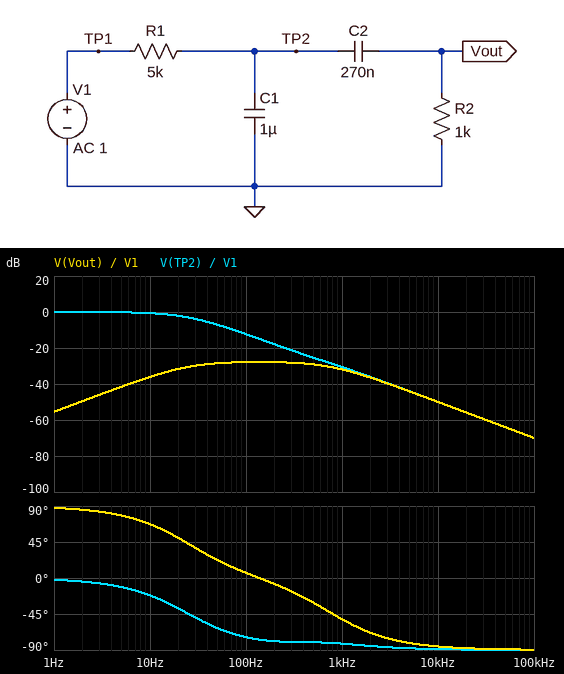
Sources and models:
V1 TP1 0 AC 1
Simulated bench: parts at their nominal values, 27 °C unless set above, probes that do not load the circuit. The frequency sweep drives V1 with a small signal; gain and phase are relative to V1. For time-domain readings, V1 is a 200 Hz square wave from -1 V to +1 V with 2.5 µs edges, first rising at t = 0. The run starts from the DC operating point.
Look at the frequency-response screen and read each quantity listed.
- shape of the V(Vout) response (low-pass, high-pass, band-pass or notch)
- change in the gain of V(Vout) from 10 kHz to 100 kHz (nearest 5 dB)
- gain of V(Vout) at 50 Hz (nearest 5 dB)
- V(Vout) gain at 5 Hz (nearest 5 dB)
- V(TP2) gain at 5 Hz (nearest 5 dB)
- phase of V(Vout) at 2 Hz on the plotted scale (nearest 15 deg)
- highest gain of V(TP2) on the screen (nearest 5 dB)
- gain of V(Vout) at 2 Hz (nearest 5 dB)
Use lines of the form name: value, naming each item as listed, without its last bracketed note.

shape of the V(Vout) response: band-pass
change in the gain of V(Vout) from 10 kHz to 100 kHz: -20 dB
gain of V(Vout) at 50 Hz: -30 dB
V(Vout) gain at 5 Hz: -40 dB
V(TP2) gain at 5 Hz: 0 dB
phase of V(Vout) at 2 Hz on the plotted scale: 90 deg
highest gain of V(TP2) on the screen: 0 dB
gain of V(Vout) at 2 Hz: -50 dB
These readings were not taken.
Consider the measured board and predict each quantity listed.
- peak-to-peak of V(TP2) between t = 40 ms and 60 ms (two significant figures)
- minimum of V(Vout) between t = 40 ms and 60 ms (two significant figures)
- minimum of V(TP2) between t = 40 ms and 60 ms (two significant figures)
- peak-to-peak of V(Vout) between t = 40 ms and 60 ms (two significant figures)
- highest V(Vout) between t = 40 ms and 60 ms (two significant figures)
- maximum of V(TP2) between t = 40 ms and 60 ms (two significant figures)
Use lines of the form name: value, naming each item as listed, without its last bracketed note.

peak-to-peak of V(TP2) between t = 40 ms and 60 ms: 400 mV
minimum of V(Vout) between t = 40 ms and 60 ms: -44 mV
minimum of V(TP2) between t = 40 ms and 60 ms: -200 mV
peak-to-peak of V(Vout) between t = 40 ms and 60 ms: 88 mV
highest V(Vout) between t = 40 ms and 60 ms: 44 mV
maximum of V(TP2) between t = 40 ms and 60 ms: 200 mV
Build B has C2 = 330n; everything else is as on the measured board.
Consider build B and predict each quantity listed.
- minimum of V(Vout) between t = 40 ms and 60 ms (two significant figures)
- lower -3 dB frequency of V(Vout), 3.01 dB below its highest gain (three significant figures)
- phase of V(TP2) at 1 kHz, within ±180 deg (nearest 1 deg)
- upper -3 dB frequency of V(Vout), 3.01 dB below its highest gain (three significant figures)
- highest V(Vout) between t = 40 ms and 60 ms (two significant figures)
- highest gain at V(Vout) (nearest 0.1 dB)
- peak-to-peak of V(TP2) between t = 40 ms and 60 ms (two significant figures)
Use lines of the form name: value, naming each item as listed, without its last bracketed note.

minimum of V(Vout) between t = 40 ms and 60 ms: -50 mV
lower -3 dB frequency of V(Vout), 3.01 dB below its highest gain: 22.1 Hz
phase of V(TP2) at 1 kHz, within ±180 deg: -81 deg
upper -3 dB frequency of V(Vout), 3.01 dB below its highest gain: 695 Hz
highest V(Vout) between t = 40 ms and 60 ms: 50 mV
highest gain at V(Vout): -26.5 dB
peak-to-peak of V(TP2) between t = 40 ms and 60 ms: 390 mV
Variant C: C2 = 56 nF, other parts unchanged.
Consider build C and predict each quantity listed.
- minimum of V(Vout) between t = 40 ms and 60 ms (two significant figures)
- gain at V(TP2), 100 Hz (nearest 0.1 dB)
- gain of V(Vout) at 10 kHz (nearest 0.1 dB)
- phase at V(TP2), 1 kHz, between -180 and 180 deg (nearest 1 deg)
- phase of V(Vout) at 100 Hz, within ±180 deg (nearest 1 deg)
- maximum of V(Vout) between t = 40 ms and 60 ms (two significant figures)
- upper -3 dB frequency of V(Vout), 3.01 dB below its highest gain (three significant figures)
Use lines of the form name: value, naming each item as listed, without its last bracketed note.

minimum of V(Vout) between t = 40 ms and 60 ms: -12 mV
gain at V(TP2), 100 Hz: -10.8 dB
gain of V(Vout) at 10 kHz: -50.3 dB
phase at V(TP2), 1 kHz, between -180 and 180 deg: -87 deg
phase of V(Vout) at 100 Hz, within ±180 deg: 15 deg
maximum of V(Vout) between t = 40 ms and 60 ms: 12 mV
upper -3 dB frequency of V(Vout), 3.01 dB below its highest gain: 3.06 kHz
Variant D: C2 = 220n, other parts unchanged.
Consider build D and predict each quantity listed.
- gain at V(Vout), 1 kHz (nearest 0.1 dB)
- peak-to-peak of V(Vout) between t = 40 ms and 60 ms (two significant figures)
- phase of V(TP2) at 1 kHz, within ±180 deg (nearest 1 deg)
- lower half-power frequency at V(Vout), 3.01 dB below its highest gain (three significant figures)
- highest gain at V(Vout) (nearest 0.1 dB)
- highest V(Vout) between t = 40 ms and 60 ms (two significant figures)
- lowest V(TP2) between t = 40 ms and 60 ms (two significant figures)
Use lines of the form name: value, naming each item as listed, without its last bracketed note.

gain at V(Vout), 1 kHz: -32.5 dB
peak-to-peak of V(Vout) between t = 40 ms and 60 ms: 76 mV
phase of V(TP2) at 1 kHz, within ±180 deg: -83 deg
lower half-power frequency at V(Vout), 3.01 dB below its highest gain: 24.5 Hz
highest gain at V(Vout): -29.2 dB
highest V(Vout) between t = 40 ms and 60 ms: 38 mV
lowest V(TP2) between t = 40 ms and 60 ms: -210 mV
